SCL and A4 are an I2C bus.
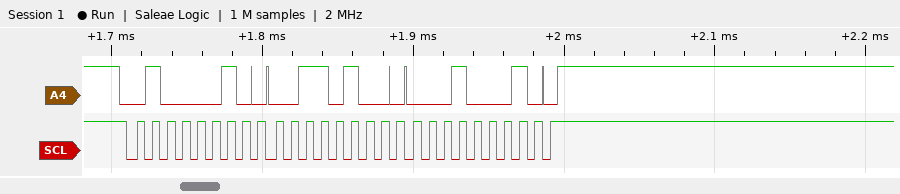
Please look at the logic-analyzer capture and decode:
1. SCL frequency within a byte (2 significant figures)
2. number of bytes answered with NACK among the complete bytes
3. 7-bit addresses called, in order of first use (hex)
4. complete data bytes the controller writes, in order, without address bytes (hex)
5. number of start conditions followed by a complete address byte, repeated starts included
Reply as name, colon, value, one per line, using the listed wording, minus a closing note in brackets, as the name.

SCL frequency within a byte: 100 kHz
number of bytes answered with NACK among the complete bytes: 0
7-bit addresses called, in order of first use: 0x21
complete data bytes the controller writes, in order, without address bytes: 34 11
number of start conditions followed by a complete address byte, repeated starts included: 1
